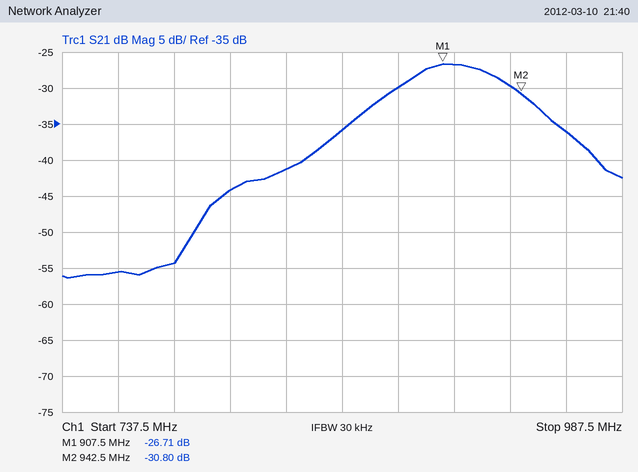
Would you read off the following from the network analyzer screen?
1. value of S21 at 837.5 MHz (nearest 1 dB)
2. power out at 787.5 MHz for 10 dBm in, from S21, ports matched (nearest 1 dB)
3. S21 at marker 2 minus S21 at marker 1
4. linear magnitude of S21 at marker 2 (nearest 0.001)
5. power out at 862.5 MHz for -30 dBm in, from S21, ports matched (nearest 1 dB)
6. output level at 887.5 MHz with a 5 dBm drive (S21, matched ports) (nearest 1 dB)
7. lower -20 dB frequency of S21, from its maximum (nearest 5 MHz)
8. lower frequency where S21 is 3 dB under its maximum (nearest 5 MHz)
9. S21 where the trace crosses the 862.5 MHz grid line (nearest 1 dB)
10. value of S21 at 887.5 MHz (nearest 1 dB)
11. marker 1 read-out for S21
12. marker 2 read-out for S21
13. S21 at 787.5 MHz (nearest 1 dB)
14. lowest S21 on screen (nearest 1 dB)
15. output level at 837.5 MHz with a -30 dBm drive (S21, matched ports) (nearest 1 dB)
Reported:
-41 dB
-44 dBm
-4.09 dB
0.029
-66 dBm
-25 dBm
805 MHz
890 MHz
-36 dB
-30 dB
-26.71 dB
-30.80 dB
-54 dB
-56 dB
-71 dBm
